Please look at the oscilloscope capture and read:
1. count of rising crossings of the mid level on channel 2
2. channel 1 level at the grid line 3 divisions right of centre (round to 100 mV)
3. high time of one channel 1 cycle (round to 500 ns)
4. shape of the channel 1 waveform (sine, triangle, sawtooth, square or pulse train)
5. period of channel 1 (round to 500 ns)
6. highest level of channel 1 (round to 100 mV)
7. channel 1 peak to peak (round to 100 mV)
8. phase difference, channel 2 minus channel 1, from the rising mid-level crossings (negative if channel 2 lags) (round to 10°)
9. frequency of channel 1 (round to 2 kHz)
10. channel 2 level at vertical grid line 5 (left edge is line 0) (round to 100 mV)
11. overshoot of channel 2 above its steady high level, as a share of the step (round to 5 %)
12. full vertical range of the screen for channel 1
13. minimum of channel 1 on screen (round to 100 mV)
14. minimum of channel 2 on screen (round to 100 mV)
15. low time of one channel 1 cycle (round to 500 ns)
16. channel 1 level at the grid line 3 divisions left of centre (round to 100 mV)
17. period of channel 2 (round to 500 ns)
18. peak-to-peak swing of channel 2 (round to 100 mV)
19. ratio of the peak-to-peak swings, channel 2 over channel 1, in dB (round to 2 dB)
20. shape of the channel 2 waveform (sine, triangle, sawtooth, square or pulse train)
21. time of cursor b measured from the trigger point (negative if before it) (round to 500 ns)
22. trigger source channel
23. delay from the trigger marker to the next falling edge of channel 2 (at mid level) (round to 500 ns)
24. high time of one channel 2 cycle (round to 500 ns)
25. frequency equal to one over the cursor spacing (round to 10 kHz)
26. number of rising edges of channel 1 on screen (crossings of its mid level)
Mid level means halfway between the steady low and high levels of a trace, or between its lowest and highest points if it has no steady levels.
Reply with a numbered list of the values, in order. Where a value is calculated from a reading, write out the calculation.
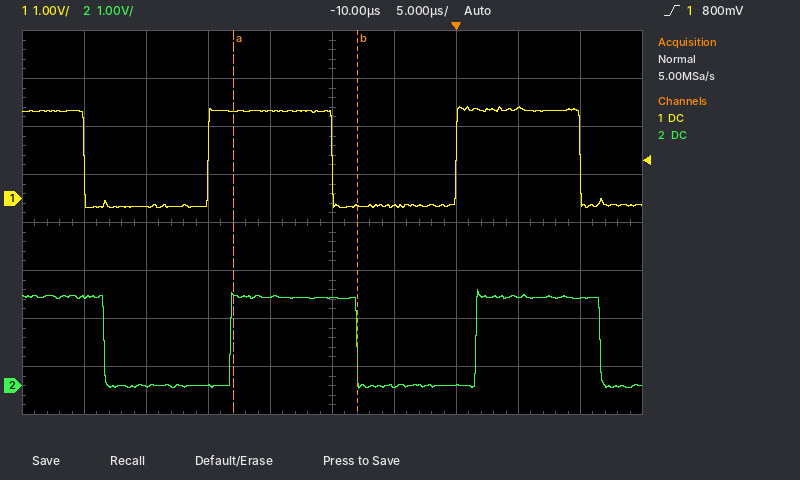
1. 2
2. 1.9 V
3. 10.0 µs
4. square
5. 20.0 µs
6. 1.9 V
7. 1.9 V − (-200 mV) = 2.1 V
8. −360° × (+1.5 µs) / 20.0 µs ≈ -27.0°, so -30° to the nearest 10°
9. 1 / 20.0 µs ≈ 50 kHz
10. 1.8 V
11. 10 %
12. 8 V
13. -200 mV
14. -100 mV
15. 10.0 µs
16. -200 mV
17. 20.0 µs
18. 2.0 V − (-100 mV) = 2.1 V
19. 20 log10(2.1 V / 2.1 V) ≈ 0 dB
20. square
21. -8.0 µs
22. channel 1
23. 11.5 µs
24. 10.0 µs
25. 1 / 10.0 µs ≈ 100 kHz
26. 2
